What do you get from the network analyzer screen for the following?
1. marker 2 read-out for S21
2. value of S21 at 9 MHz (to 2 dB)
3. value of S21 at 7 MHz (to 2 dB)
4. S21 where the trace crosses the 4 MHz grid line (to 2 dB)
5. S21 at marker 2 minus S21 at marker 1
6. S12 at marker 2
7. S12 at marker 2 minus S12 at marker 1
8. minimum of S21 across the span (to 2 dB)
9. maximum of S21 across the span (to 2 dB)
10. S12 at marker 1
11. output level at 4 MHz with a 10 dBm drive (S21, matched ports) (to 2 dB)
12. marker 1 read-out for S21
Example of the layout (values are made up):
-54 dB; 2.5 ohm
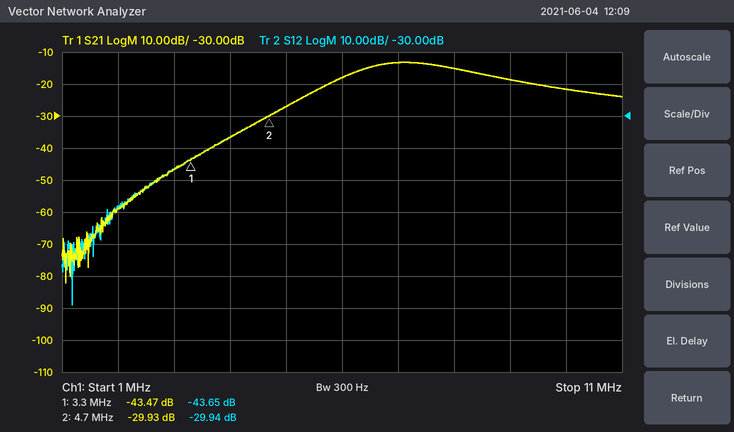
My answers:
-29.93 dB; -18 dB; -14 dB; -36 dB; 13.54 dB; -29.94 dB; 13.71 dB; -82 dB; -14 dB; -43.65 dB; -26 dBm; -43.47 dB
